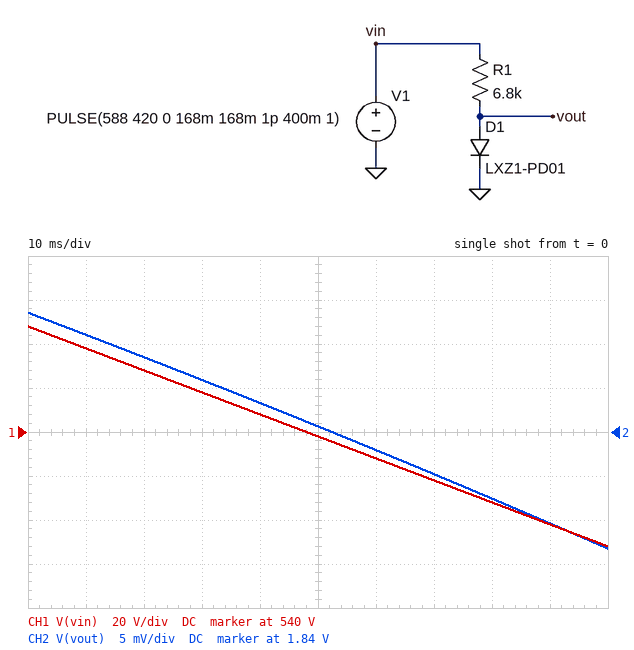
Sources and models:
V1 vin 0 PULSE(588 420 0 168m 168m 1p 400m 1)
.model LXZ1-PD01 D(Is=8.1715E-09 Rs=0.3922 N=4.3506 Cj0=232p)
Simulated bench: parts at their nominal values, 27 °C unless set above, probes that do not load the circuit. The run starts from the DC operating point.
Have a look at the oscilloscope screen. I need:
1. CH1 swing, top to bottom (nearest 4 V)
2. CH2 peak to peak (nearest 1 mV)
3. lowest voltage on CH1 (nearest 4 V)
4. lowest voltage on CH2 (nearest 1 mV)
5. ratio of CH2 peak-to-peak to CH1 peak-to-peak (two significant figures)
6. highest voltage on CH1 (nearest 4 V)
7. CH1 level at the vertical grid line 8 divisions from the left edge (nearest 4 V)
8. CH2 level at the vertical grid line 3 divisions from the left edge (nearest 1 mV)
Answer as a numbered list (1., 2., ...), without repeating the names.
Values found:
1. 100 V
2. 27 mV
3. 488 V
4. 1.827 V
5. 0.00027
6. 588 V
7. 508 V
8. 1.846 V
